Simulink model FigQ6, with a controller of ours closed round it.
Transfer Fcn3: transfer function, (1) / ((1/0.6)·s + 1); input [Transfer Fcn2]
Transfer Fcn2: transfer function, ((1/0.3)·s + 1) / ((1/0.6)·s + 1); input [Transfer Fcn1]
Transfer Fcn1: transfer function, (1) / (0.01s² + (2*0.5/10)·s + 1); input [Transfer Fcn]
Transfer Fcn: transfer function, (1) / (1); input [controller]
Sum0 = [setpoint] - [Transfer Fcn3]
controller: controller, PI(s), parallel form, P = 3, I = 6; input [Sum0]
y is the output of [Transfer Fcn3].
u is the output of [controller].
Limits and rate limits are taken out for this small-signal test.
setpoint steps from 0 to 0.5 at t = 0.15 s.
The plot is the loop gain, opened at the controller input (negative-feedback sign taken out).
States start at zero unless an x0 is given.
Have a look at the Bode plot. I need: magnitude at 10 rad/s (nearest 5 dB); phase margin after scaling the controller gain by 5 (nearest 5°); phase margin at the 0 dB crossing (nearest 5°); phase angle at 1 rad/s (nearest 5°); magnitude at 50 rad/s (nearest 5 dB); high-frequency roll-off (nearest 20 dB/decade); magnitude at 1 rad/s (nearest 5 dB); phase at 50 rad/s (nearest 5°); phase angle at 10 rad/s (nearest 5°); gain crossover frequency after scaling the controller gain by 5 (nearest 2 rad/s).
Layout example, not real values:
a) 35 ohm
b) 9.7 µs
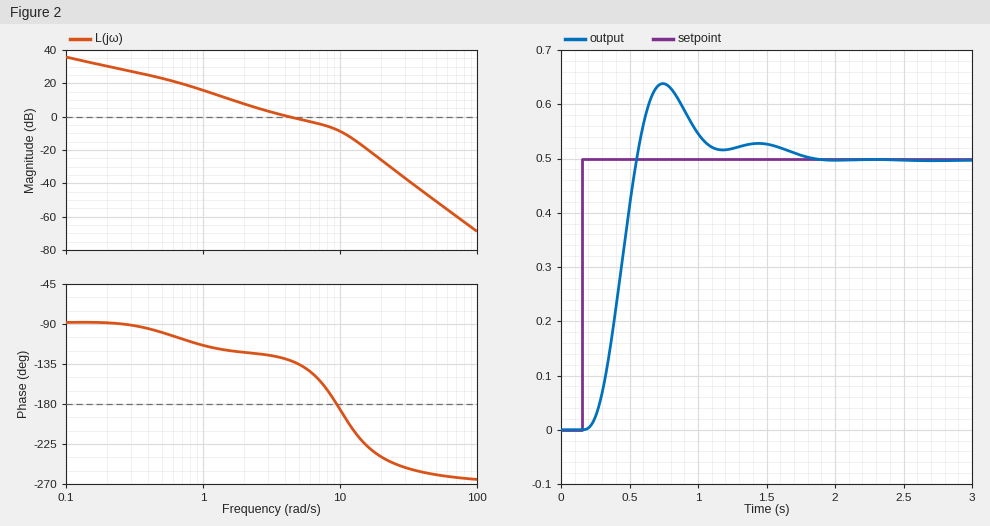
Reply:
a) -10 dB
b) -30°
c) 50°
d) -115°
e) -50 dB
f) -60 dB/decade
g) 15 dB
h) -260°
i) -185°
j) 12 rad/s
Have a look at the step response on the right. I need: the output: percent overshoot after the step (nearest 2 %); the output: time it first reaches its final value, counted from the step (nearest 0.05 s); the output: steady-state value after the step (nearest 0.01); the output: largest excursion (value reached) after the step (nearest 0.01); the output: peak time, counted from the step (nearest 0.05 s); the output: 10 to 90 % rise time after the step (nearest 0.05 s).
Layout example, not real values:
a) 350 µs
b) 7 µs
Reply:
a) 28 %
b) 0.40 s
c) 0.50
d) 0.64
e) 0.60 s
f) 0.25 s
